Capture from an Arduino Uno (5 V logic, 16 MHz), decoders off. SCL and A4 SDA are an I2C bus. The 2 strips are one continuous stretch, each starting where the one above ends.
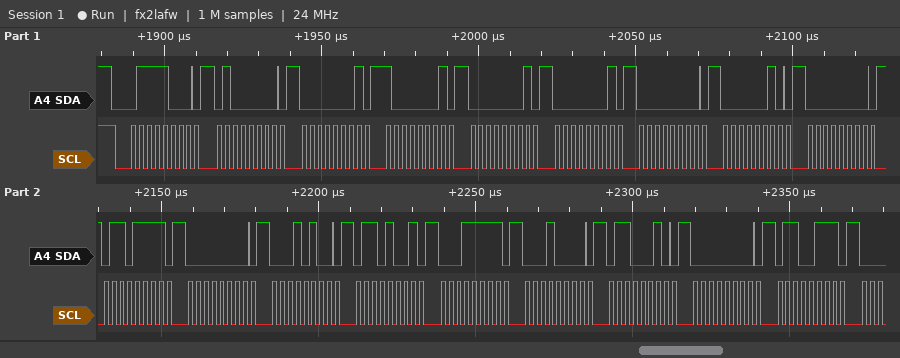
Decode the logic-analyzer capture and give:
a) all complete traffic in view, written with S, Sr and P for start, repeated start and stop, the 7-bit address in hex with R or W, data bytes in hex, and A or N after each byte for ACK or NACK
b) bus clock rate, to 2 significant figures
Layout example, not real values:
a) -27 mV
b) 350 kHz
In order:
a) S 3CW A 40 A 01 A 81 A 01 A 01 A 00 A 02 A 00 A 6F A 00 A 14 A 69 A 1F A 10 A 62 A 00 A 67 A
b) 400 kHz
